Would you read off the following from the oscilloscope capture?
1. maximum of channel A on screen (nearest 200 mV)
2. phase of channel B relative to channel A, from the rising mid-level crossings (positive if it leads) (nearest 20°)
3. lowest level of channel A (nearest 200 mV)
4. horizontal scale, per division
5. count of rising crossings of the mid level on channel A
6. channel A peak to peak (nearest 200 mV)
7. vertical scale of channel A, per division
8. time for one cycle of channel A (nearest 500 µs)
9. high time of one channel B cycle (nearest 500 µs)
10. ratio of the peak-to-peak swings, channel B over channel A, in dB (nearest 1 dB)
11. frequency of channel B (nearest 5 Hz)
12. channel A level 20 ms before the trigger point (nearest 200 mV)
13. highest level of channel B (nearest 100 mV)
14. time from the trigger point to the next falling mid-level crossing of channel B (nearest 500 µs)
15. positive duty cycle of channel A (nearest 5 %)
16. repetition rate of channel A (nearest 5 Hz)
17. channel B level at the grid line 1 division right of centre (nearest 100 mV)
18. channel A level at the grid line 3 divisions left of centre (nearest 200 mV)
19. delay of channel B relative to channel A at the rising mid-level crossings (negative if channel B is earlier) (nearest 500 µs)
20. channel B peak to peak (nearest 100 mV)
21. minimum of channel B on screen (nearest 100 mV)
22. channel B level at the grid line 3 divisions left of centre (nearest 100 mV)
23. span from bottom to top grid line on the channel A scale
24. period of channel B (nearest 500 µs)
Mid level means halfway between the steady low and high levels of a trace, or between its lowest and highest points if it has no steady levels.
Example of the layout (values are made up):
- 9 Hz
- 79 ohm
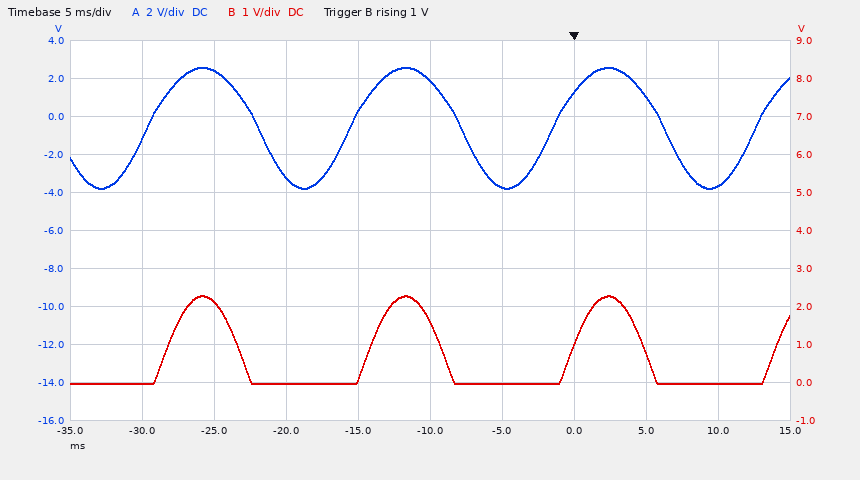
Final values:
- 2.6 V
- -40°
- -3.8 V
- 5 ms
- 4
- 6.4 V
- 2 V
- 14.0 ms
- 4.5 ms
- -9 dB
- 70 Hz
- -3.2 V
- 2.3 V
- 4.5 ms
- 55 %
- 70 Hz
- 0.0 V
- 2.4 V
- +1.5 ms
- 2.3 V
- 0.0 V
- 2.1 V
- 20 V
- 14.0 ms
